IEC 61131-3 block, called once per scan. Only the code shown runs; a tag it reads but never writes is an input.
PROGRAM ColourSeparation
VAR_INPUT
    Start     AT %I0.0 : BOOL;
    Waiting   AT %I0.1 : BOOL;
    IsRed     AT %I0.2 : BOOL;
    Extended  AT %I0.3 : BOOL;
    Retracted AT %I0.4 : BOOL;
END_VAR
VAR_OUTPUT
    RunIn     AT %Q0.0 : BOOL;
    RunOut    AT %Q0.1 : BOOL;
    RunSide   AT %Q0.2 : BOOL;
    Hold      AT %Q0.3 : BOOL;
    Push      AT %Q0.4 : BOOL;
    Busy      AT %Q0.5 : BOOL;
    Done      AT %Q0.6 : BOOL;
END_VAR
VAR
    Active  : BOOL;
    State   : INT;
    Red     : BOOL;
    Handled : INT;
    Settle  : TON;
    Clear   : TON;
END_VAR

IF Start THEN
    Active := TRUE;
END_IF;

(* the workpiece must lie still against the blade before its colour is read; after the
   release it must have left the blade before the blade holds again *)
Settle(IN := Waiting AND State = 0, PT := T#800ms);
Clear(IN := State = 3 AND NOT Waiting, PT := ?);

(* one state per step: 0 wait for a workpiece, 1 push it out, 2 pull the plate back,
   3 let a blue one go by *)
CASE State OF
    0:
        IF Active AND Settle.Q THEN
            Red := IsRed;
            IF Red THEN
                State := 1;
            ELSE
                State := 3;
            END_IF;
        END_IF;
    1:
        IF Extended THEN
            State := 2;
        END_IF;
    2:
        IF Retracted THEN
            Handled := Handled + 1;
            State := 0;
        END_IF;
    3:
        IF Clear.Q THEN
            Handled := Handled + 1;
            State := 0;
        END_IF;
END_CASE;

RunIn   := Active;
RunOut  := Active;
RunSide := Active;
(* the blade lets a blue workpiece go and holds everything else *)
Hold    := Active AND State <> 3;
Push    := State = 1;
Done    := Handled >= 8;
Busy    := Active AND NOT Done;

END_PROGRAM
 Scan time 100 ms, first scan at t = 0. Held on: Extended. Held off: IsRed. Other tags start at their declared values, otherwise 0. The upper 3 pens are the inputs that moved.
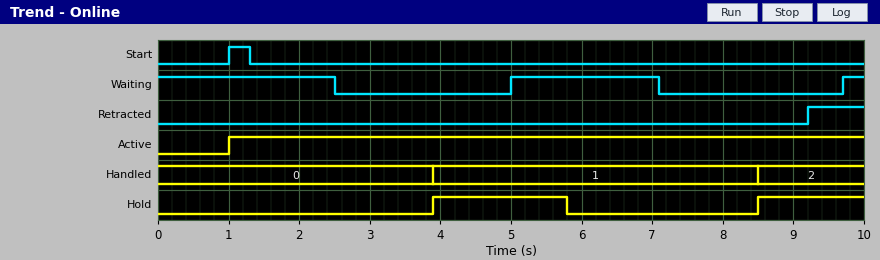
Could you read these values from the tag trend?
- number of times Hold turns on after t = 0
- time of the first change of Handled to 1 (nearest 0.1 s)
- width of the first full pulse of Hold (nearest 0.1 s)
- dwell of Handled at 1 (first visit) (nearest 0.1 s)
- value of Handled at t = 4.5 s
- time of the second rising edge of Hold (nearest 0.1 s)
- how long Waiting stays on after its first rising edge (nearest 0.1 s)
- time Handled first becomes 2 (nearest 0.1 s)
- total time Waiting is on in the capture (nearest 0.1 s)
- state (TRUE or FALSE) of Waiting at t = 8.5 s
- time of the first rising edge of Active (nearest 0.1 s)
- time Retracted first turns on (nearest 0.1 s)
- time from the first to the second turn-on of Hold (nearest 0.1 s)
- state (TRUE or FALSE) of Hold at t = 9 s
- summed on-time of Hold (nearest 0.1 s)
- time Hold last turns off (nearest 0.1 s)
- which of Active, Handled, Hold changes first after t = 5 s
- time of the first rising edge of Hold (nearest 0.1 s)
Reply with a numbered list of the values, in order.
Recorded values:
1. 2
2. 3.9 s
3. 1.9 s
4. 4.6 s
5. 1
6. 8.5 s
7. 2.1 s
8. 8.5 s
9. 4.9 s
10. FALSE
11. 1.0 s
12. 9.2 s
13. 4.6 s
14. TRUE
15. 3.4 s
16. 5.8 s
17. Hold
18. 3.9 s
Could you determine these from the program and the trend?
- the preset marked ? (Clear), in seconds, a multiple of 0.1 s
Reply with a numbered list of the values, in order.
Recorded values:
1. 1.4 s
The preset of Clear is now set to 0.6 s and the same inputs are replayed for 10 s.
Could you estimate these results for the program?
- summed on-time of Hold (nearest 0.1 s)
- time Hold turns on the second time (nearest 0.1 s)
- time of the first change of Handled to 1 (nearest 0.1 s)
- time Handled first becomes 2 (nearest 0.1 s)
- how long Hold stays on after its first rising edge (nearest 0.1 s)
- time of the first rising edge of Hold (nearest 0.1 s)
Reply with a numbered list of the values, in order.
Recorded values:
1. 5.0 s
2. 7.7 s
3. 3.1 s
4. 7.7 s
5. 2.7 s
6. 3.1 s
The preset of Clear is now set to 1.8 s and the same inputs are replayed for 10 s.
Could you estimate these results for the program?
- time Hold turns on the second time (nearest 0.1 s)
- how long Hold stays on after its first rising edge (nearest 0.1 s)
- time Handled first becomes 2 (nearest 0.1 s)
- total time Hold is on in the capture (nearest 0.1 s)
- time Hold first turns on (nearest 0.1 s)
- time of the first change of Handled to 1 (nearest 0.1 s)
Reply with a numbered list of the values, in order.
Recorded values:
1. 8.9 s
2. 1.5 s
3. 8.9 s
4. 2.6 s
5. 4.3 s
6. 4.3 s
